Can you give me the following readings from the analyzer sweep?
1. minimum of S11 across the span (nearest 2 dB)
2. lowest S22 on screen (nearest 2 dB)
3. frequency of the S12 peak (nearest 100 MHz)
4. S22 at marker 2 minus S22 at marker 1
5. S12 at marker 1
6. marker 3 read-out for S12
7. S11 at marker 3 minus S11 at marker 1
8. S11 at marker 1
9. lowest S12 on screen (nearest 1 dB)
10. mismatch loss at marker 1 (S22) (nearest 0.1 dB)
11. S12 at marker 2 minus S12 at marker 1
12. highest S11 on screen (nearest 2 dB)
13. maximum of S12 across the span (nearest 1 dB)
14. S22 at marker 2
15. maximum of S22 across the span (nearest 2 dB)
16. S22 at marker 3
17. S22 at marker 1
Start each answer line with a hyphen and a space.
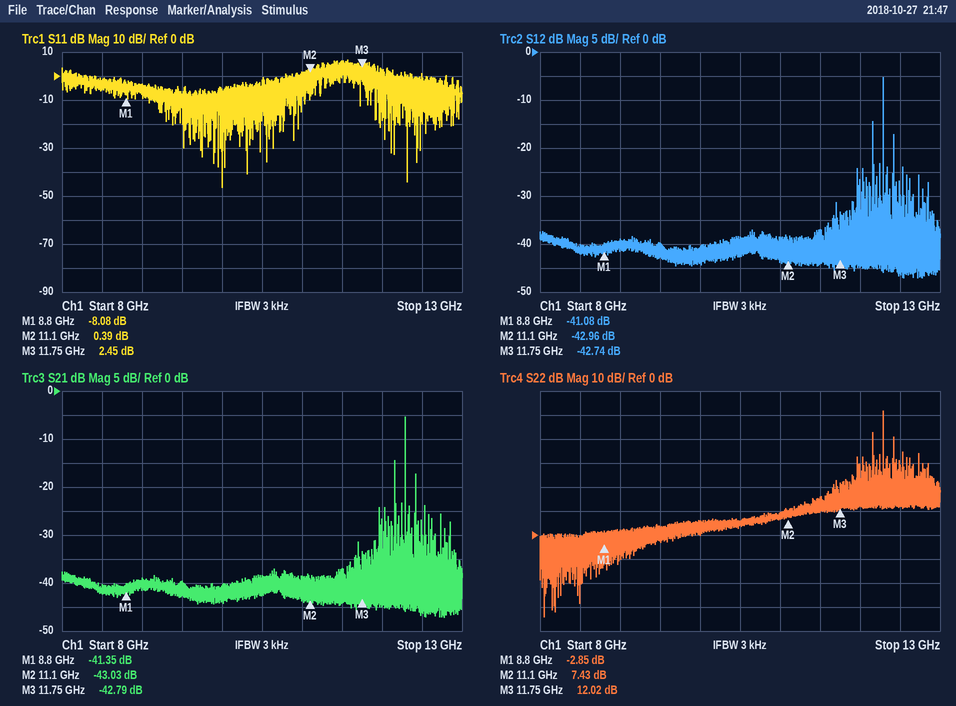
- -46 dB
- -34 dB
- 12.3 GHz
- 10.28 dB
- -41.08 dB
- -42.74 dB
- 10.53 dB
- -8.08 dB
- -47 dB
- 3.2 dB
- -1.88 dB
- 6 dB
- -5 dB
- 7.43 dB
- 52 dB
- 12.02 dB
- -2.85 dB
